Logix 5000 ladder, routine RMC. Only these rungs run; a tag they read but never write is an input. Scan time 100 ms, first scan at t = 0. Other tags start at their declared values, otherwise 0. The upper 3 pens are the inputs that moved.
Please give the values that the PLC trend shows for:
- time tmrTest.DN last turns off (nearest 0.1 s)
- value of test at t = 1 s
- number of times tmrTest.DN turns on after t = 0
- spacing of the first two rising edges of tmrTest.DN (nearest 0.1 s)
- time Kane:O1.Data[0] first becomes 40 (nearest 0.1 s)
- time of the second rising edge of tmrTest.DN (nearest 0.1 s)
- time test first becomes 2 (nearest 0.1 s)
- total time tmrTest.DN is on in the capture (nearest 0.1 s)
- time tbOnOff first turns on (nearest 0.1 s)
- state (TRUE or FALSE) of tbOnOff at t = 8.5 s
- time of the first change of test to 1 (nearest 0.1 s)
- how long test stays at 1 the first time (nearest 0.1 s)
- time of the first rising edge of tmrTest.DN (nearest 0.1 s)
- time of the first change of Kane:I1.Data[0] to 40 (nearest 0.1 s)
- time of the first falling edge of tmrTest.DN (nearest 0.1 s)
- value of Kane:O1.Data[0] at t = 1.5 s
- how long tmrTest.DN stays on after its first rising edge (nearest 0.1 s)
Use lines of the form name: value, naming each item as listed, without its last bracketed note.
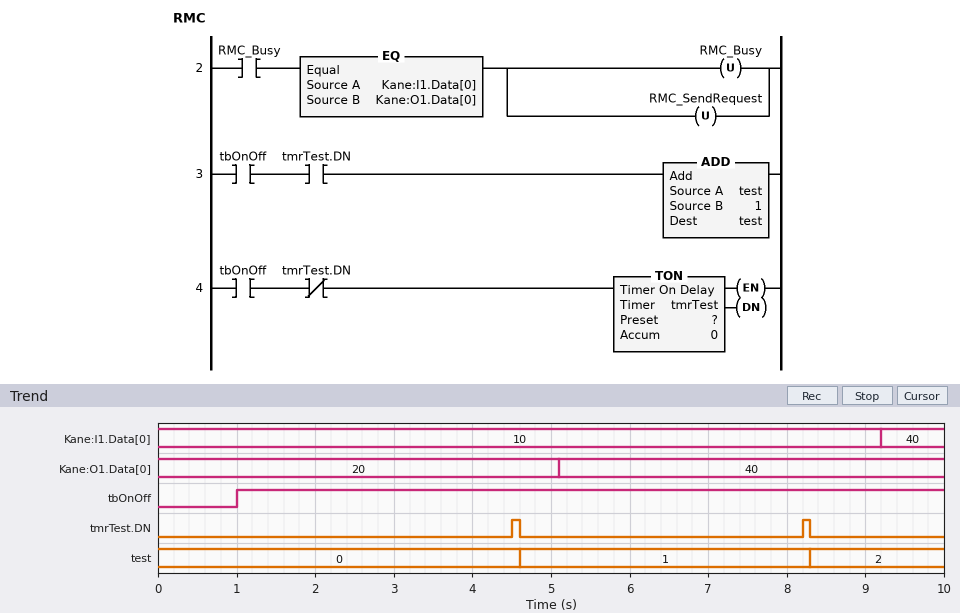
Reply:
time tmrTest.DN last turns off: 8.3 s
value of test at t = 1 s: 0
number of times tmrTest.DN turns on after t = 0: 2
spacing of the first two rising edges of tmrTest.DN: 3.7 s
time Kane:O1.Data[0] first becomes 40: 5.1 s
time of the second rising edge of tmrTest.DN: 8.2 s
time test first becomes 2: 8.3 s
total time tmrTest.DN is on in the capture: 0.2 s
time tbOnOff first turns on: 1.0 s
state (TRUE or FALSE) of tbOnOff at t = 8.5 s: TRUE
time of the first change of test to 1: 4.6 s
how long test stays at 1 the first time: 3.7 s
time of the first rising edge of tmrTest.DN: 4.5 s
time of the first change of Kane:I1.Data[0] to 40: 9.2 s
time of the first falling edge of tmrTest.DN: 4.6 s
value of Kane:O1.Data[0] at t = 1.5 s: 20
how long tmrTest.DN stays on after its first rising edge: 0.1 s
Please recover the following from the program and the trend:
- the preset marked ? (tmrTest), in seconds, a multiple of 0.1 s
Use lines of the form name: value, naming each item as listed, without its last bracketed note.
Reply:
the preset marked ? (tmrTest), in seconds, a multiple of 0.1 s: 3.5 s
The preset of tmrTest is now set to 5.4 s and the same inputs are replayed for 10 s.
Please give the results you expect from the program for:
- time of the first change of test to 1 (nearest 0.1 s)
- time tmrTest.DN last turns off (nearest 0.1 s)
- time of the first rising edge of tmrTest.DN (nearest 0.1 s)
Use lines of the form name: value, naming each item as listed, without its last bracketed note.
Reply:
time of the first change of test to 1: 6.5 s
time tmrTest.DN last turns off: 6.5 s
time of the first rising edge of tmrTest.DN: 6.4 s
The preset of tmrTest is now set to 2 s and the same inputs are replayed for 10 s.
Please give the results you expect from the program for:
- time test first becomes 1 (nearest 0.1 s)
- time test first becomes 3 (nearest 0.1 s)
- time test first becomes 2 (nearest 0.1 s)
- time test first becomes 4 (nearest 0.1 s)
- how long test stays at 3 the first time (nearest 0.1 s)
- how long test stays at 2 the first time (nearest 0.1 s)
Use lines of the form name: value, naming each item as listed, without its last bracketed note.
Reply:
time test first becomes 1: 3.1 s
time test first becomes 3: 7.5 s
time test first becomes 2: 5.3 s
time test first becomes 4: 9.7 s
how long test stays at 3 the first time: 2.2 s
how long test stays at 2 the first time: 2.2 s
